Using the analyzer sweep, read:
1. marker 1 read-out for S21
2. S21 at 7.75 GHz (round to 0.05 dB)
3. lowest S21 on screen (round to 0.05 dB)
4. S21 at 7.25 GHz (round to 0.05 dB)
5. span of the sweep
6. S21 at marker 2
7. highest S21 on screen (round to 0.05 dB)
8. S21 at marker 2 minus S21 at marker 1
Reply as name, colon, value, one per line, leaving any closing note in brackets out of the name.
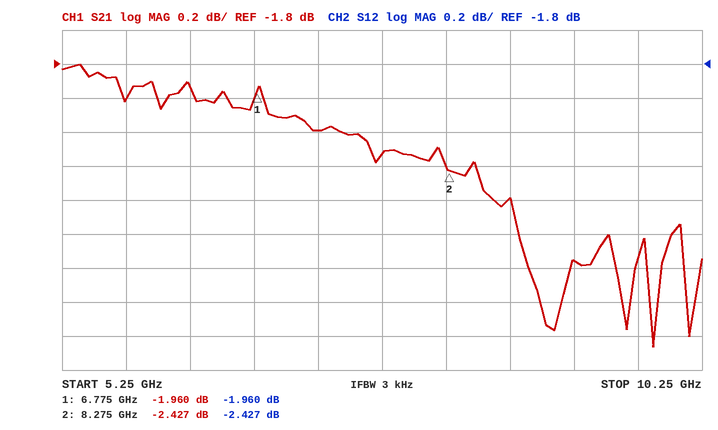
marker 1 read-out for S21: -1.960 dB
S21 at 7.75 GHz: -2.35 dB
lowest S21 on screen: -3.45 dB
S21 at 7.25 GHz: -2.20 dB
span of the sweep: 5 GHz
S21 at marker 2: -2.427 dB
highest S21 on screen: -1.80 dB
S21 at marker 2 minus S21 at marker 1: -0.467 dB
